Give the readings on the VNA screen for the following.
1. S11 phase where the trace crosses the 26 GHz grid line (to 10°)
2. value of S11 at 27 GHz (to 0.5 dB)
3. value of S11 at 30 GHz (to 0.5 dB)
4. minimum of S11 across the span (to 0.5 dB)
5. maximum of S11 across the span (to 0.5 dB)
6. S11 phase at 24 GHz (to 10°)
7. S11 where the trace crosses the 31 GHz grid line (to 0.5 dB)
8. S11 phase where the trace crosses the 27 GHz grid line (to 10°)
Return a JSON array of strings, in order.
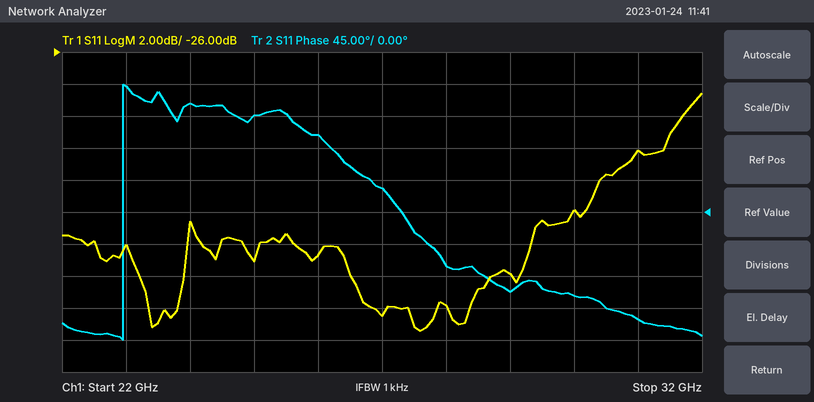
["110°", "-42.5 dB", "-36.0 dB", "-43.5 dB", "-28.5 dB", "150°", "-32.0 dB", "30°"]
